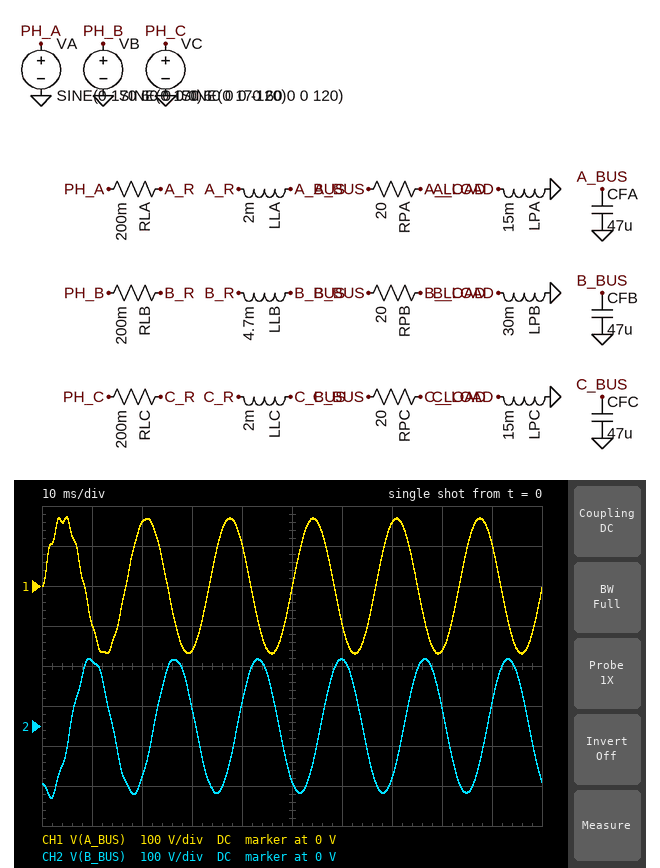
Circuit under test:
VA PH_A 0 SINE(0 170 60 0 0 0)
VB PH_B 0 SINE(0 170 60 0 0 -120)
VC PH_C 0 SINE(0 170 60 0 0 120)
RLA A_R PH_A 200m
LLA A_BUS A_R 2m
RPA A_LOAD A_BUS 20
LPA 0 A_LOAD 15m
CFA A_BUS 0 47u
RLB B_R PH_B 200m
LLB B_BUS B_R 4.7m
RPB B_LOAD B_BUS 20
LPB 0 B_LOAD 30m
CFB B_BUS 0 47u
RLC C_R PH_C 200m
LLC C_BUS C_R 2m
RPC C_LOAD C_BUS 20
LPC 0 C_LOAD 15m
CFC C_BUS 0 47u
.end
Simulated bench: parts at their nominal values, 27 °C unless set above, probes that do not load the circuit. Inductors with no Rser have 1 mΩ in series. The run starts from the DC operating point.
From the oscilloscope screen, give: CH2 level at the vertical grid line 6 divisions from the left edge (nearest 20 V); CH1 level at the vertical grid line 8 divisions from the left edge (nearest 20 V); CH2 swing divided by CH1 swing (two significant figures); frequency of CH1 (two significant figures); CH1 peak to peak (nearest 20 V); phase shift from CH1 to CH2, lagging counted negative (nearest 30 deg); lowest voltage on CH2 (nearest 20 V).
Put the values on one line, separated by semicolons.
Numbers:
160 V; -160 V; 1.0; 60 Hz; 340 V; -120 deg; -180 V
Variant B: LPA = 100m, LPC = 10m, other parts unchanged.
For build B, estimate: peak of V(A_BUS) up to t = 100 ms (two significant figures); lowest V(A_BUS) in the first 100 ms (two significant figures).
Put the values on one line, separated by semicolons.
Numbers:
180 V; -180 V
